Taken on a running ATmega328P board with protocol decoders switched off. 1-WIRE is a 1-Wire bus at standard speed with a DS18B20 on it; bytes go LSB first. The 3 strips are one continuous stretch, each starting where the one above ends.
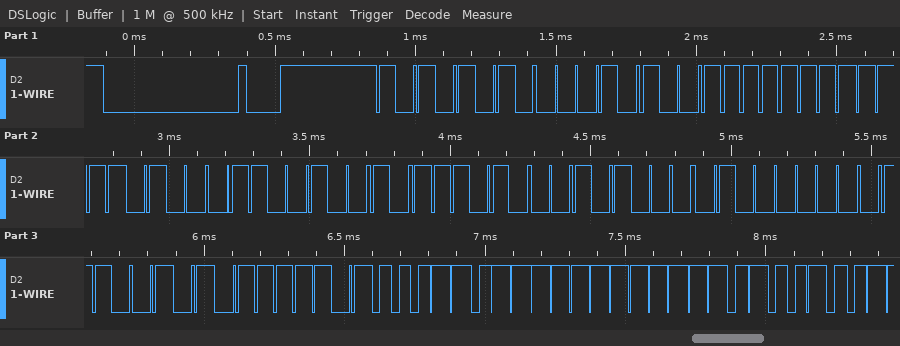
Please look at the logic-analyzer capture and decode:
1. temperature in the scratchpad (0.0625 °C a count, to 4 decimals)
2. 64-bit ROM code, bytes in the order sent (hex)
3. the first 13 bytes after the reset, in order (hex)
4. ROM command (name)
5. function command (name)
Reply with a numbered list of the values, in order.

1. -2.5000 °C
2. 28 FF 2F 26 5D 14 02 A6
3. 55 28 FF 2F 26 5D 14 02 A6 BE D8 FF 4B
4. Match ROM
5. Read Scratchpad
